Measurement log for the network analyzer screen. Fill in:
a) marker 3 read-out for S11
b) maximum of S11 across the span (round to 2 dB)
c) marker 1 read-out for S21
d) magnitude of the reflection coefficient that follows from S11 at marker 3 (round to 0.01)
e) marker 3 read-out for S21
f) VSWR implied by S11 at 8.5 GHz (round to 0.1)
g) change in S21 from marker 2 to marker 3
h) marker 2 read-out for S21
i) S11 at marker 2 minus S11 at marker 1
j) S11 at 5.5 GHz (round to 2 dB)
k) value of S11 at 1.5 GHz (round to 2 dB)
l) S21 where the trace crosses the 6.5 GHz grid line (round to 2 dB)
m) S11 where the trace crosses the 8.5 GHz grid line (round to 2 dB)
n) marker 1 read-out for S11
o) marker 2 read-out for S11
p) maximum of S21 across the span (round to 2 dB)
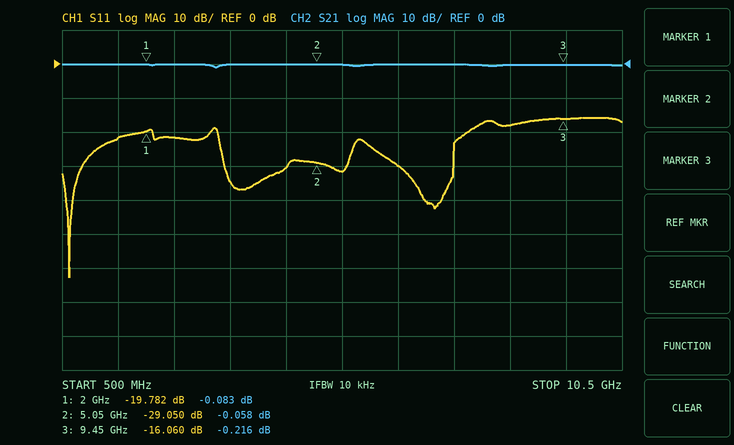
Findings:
-16.060 dB
-16 dB
-0.083 dB
0.16
-0.216 dB
1.3
-0.158 dB
-0.058 dB
-9.268 dB
-32 dB
-22 dB
0 dB
-18 dB
-19.782 dB
-29.050 dB
0 dB
